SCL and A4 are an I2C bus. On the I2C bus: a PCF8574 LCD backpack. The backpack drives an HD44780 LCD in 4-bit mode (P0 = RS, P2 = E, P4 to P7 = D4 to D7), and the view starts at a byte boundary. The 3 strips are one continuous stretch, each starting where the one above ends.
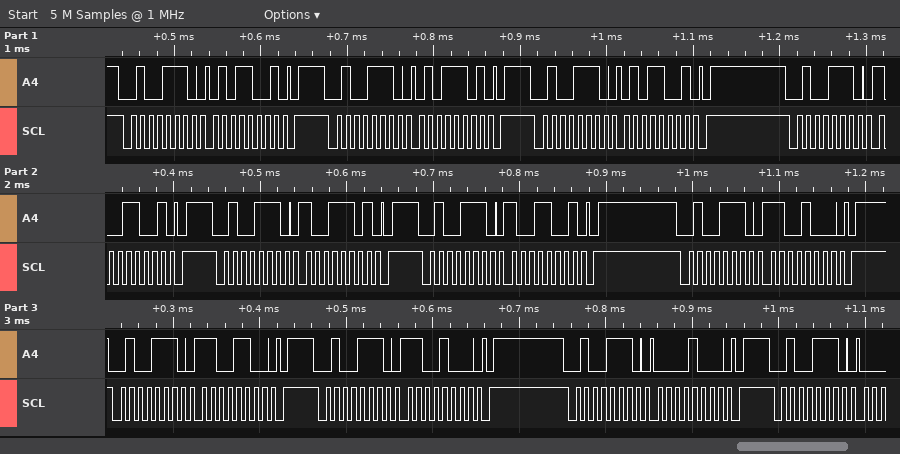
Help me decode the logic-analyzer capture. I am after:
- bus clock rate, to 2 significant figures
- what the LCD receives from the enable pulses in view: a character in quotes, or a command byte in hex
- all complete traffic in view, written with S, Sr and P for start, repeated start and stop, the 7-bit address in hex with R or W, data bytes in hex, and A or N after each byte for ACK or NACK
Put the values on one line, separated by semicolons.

100 kHz; 'Y'; S 27W A 59 A P S 27W A 5D A P S 27W A 59 A P S 27W A 99 A P S 27W A 9D A P S 27W A 99 A P S 27W A C8 A P S 27W A CC A P S 27W A C8 A P S 27W A 08 A P S 27W A
